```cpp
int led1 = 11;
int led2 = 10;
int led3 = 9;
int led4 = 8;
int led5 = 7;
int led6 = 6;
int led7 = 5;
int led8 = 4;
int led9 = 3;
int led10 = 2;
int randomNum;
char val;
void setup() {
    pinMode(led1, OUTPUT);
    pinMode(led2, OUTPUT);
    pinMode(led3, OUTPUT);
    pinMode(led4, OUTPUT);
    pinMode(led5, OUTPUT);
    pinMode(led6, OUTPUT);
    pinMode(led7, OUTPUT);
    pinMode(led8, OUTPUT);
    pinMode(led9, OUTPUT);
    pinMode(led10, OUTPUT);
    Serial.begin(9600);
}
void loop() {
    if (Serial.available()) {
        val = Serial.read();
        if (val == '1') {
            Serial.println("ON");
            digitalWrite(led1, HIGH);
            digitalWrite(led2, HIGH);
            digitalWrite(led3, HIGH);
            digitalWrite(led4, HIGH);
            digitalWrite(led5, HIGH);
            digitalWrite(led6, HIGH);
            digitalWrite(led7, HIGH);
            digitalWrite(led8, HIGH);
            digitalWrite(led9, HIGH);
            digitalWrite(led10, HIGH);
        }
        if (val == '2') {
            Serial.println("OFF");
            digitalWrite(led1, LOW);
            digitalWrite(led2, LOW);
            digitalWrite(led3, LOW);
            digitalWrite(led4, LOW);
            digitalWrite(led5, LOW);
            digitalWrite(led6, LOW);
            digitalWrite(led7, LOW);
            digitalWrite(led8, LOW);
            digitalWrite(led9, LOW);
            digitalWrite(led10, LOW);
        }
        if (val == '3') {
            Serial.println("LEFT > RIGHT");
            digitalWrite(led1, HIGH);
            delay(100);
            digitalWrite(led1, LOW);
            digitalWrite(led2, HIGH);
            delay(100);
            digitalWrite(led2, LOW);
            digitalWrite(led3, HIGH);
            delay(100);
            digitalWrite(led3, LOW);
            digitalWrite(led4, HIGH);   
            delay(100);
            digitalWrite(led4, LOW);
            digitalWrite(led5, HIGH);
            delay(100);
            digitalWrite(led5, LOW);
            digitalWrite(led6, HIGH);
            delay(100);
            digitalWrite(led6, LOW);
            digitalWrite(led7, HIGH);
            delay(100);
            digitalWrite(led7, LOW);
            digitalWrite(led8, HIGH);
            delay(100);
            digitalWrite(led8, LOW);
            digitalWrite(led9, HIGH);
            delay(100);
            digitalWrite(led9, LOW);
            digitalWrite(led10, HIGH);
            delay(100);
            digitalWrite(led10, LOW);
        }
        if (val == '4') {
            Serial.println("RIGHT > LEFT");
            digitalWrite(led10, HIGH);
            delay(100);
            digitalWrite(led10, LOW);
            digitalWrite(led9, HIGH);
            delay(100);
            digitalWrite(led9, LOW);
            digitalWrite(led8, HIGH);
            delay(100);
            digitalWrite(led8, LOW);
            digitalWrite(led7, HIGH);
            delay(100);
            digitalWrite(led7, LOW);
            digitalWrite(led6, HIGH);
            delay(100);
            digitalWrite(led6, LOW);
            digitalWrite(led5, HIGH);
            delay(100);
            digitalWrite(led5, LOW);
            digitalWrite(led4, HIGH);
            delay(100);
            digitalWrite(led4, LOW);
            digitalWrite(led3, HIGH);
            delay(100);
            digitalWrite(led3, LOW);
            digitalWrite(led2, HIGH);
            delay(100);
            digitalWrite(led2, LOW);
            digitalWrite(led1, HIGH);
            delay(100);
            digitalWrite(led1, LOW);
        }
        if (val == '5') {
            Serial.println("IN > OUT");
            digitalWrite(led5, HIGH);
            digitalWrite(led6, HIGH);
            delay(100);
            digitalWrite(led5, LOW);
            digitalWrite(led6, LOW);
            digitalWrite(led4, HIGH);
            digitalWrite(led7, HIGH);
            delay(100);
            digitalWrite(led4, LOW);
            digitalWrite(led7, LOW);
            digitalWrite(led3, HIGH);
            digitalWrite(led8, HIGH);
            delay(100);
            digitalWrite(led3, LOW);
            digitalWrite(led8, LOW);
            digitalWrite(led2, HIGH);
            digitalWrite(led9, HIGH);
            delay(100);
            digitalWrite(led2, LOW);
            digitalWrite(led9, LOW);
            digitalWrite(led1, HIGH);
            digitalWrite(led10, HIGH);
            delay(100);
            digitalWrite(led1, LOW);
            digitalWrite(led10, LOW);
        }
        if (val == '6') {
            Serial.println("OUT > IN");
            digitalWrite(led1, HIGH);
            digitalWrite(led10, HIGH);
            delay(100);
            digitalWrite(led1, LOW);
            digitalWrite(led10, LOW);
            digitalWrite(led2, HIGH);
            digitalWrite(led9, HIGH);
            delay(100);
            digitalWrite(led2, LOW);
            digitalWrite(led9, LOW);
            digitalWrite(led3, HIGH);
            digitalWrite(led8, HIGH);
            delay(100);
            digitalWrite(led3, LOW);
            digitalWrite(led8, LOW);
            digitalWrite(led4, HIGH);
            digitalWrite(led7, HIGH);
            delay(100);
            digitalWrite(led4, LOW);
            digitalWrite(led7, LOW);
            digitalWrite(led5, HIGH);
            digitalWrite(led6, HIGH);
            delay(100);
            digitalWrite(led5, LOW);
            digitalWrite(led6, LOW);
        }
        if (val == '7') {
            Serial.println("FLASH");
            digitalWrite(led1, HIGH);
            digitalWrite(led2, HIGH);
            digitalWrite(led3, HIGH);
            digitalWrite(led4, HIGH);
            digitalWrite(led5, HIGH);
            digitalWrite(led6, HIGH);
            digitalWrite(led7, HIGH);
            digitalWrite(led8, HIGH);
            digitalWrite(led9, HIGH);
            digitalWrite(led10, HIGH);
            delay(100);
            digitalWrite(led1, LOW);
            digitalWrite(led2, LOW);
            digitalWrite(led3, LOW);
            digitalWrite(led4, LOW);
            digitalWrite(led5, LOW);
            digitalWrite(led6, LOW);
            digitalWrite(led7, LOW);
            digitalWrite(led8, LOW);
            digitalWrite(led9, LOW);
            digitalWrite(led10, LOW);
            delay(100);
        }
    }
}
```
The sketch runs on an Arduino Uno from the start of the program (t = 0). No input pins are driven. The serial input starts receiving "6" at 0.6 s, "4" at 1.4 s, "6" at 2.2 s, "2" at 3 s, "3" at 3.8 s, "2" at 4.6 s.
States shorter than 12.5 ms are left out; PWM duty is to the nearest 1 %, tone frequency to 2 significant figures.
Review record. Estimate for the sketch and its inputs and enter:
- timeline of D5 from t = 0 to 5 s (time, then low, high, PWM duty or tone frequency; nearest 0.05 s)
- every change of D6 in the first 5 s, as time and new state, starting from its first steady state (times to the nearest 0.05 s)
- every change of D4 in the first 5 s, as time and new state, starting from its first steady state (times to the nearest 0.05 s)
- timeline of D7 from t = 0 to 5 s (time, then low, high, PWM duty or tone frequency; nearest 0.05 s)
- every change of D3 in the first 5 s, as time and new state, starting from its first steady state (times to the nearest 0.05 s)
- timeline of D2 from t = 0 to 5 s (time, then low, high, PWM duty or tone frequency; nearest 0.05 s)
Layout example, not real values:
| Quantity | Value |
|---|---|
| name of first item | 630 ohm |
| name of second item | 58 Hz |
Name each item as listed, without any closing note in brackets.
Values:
| Quantity | Value |
|---|---|
| timeline of D5 from t = 0 to 5 s | 0 s low; 0.9 s high; 1 s low; 1.7 s high; 1.8 s low; 2.7 s high; 2.8 s low; 4.4 s high; 4.5 s low |
| every change of D6 in the first 5 s, as time and new state, starting from its first steady state | 0 s low; 1 s high; 1.1 s low; 1.8 s high; 1.9 s low; 2.8 s high; 2.9 s low; 4.3 s high; 4.4 s low |
| every change of D4 in the first 5 s, as time and new state, starting from its first steady state | 0 s low; 0.8 s high; 0.9 s low; 1.6 s high; 1.7 s low; 2.6 s high; 2.7 s low; 4.5 s high; 4.6 s low |
| timeline of D7 from t = 0 to 5 s | 0 s low; 1 s high; 1.1 s low; 1.9 s high; 2 s low; 2.8 s high; 2.9 s low; 4.2 s high; 4.3 s low |
| every change of D3 in the first 5 s, as time and new state, starting from its first steady state | 0 s low; 0.7 s high; 0.8 s low; 1.5 s high; 1.6 s low; 2.5 s high; 2.6 s low; 4.6 s high; 4.7 s low |
| timeline of D2 from t = 0 to 5 s | 0 s low; 0.6 s high; 0.7 s low; 1.4 s high; 1.5 s low; 2.4 s high; 2.5 s low; 4.7 s high; 4.8 s low |
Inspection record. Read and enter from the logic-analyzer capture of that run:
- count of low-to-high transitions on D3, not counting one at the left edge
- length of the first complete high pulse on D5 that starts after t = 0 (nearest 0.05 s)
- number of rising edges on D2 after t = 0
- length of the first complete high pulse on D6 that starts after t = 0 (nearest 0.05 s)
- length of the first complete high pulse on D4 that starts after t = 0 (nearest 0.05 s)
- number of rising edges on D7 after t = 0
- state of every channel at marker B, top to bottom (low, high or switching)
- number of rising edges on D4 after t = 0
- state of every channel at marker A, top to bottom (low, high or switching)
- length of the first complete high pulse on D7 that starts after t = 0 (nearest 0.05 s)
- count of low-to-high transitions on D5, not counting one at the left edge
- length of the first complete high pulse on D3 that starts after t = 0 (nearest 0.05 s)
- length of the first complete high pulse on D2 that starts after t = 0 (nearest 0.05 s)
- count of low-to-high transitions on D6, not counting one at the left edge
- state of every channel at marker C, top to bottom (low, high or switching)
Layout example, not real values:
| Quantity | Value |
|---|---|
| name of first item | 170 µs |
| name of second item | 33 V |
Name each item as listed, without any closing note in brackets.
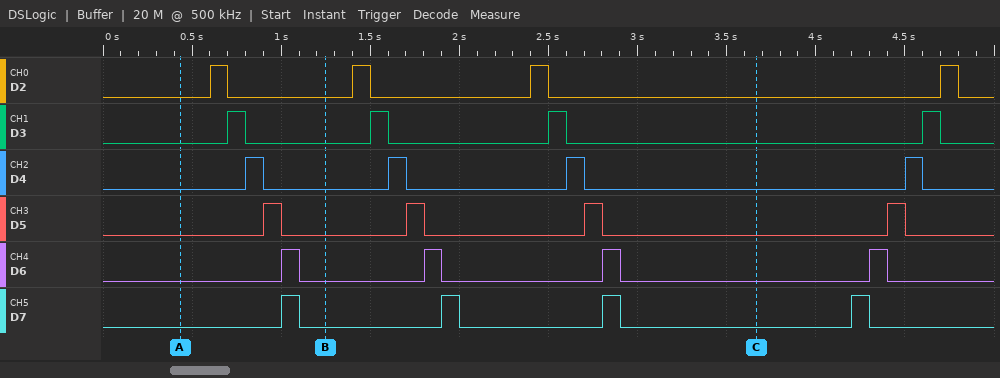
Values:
| Quantity | Value |
|---|---|
| count of low-to-high transitions on D3, not counting one at the left edge | 4 |
| length of the first complete high pulse on D5 that starts after t = 0 | 0.10 s |
| number of rising edges on D2 after t = 0 | 4 |
| length of the first complete high pulse on D6 that starts after t = 0 | 0.10 s |
| length of the first complete high pulse on D4 that starts after t = 0 | 0.10 s |
| number of rising edges on D7 after t = 0 | 4 |
| state of every channel at marker B, top to bottom | D2 low, D3 low, D4 low, D5 low, D6 low, D7 low |
| number of rising edges on D4 after t = 0 | 4 |
| state of every channel at marker A, top to bottom | D2 low, D3 low, D4 low, D5 low, D6 low, D7 low |
| length of the first complete high pulse on D7 that starts after t = 0 | 0.10 s |
| count of low-to-high transitions on D5, not counting one at the left edge | 4 |
| length of the first complete high pulse on D3 that starts after t = 0 | 0.10 s |
| length of the first complete high pulse on D2 that starts after t = 0 | 0.10 s |
| count of low-to-high transitions on D6, not counting one at the left edge | 4 |
| state of every channel at marker C, top to bottom | D2 low, D3 low, D4 low, D5 low, D6 low, D7 low |
